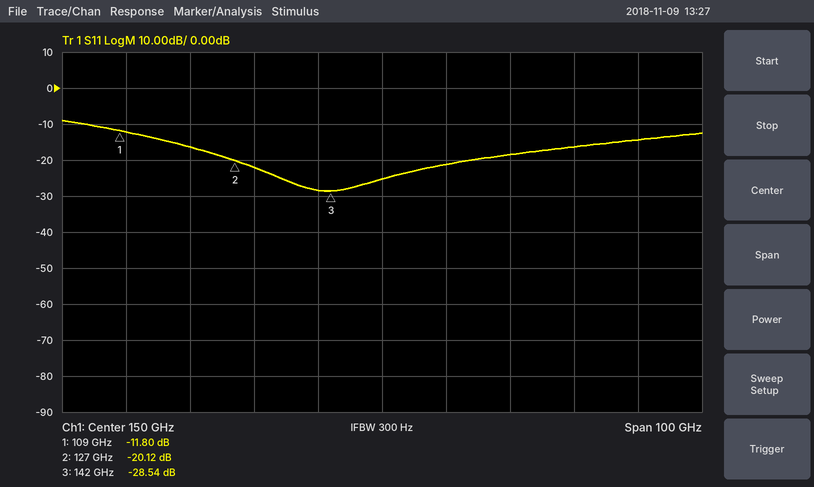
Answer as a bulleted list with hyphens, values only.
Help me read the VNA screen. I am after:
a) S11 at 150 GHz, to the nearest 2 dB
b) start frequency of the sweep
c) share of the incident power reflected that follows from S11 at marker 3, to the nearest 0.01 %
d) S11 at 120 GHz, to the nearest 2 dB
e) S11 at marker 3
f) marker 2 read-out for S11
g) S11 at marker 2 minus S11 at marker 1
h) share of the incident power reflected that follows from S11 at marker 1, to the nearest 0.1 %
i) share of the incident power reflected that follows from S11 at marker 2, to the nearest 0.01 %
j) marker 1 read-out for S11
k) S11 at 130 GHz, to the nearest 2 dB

- -26 dB
- 100 GHz
- 0.14 %
- -16 dB
- -28.54 dB
- -20.12 dB
- -8.32 dB
- 6.6 %
- 0.97 %
- -11.80 dB
- -22 dB
